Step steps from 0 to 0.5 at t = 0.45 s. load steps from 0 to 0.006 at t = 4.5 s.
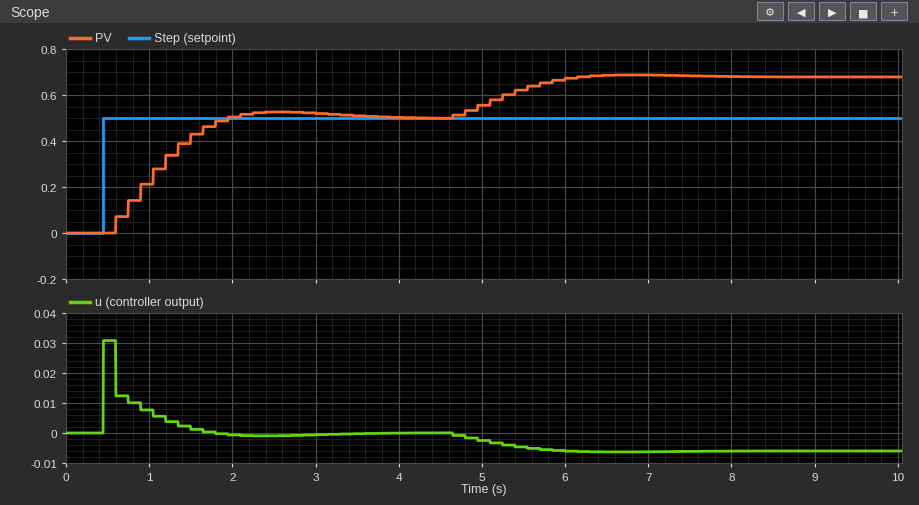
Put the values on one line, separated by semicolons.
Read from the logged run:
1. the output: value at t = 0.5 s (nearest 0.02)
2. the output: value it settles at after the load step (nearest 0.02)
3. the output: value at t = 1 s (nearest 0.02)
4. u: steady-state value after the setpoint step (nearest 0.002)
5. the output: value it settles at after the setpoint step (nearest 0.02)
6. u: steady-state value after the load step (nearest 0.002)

0.00; 0.68; 0.22; 0.000; 0.50; -0.006
